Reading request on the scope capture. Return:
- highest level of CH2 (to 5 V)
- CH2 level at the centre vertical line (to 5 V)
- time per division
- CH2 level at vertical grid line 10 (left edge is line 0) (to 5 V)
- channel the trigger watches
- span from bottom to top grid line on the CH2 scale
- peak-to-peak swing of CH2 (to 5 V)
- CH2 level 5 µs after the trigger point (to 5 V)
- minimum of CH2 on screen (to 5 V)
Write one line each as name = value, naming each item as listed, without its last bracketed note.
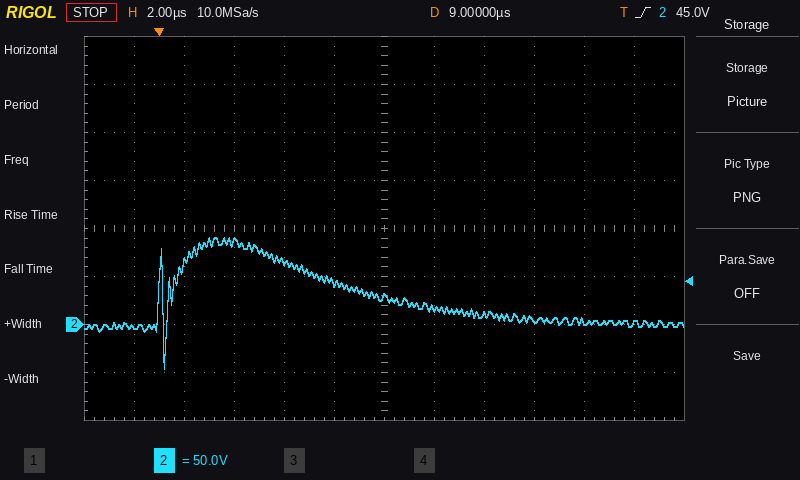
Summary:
highest level of CH2 = 90 V
CH2 level at the centre vertical line = 30 V
time per division = 2 µs
CH2 level at vertical grid line 10 (left edge is line 0) = 5 V
channel the trigger watches = CH2
span from bottom to top grid line on the CH2 scale = 400 V
peak-to-peak swing of CH2 = 135 V
CH2 level 5 µs after the trigger point = 65 V
minimum of CH2 on screen = -45 V
